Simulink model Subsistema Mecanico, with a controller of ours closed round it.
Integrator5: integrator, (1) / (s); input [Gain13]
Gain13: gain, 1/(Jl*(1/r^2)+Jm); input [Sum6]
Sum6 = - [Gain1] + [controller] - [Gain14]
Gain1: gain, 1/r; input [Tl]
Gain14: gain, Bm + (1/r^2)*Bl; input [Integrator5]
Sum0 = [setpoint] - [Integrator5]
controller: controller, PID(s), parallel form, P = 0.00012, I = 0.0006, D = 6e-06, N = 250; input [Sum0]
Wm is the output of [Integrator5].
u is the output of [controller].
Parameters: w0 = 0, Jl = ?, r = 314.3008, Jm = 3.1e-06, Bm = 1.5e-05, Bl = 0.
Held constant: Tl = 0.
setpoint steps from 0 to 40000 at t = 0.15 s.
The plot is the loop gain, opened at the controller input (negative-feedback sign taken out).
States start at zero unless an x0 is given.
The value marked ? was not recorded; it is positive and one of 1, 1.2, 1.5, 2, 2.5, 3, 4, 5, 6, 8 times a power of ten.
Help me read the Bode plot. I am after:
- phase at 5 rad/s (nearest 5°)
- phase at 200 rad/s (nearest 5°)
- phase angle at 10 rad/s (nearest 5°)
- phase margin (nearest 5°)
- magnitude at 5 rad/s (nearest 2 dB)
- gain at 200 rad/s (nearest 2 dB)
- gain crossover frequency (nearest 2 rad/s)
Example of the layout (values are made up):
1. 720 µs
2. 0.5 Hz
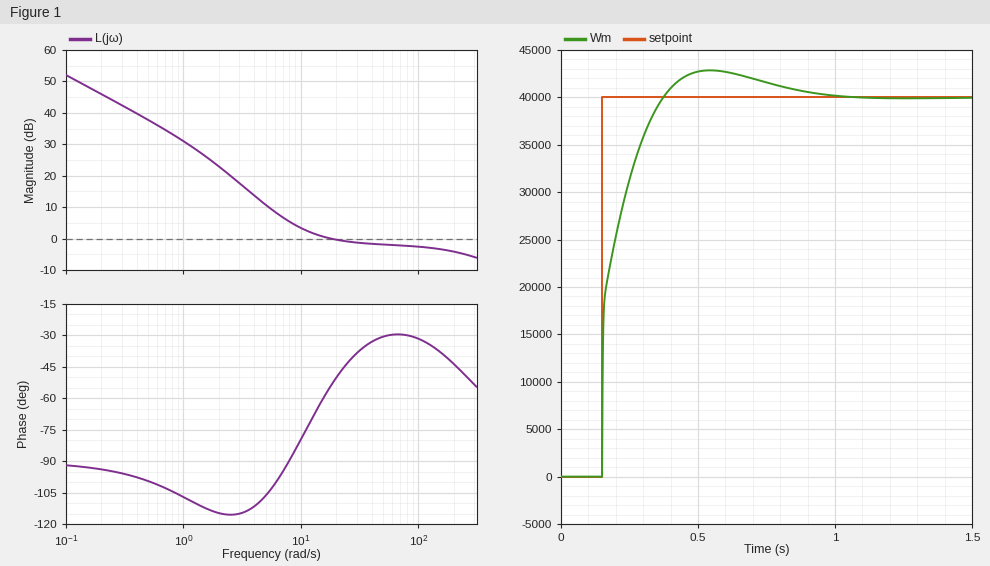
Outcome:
1. -105°
2. -45°
3. -80°
4. 125°
5. 10 dB
6. -4 dB
7. 18 rad/s
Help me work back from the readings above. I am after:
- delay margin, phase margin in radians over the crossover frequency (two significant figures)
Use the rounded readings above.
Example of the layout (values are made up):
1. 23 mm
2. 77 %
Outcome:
1. 0.12 s
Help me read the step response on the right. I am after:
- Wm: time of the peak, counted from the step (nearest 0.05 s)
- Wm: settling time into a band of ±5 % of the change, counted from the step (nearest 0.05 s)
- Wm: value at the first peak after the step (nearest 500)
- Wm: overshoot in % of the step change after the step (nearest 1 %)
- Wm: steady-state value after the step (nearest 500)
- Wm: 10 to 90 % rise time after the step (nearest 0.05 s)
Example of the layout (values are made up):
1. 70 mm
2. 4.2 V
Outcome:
1. 0.40 s
2. 0.55 s
3. 43000
4. 7 %
5. 40000
6. 0.15 s
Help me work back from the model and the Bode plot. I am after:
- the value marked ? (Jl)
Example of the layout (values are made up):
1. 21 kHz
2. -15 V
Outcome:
1. 0.5
